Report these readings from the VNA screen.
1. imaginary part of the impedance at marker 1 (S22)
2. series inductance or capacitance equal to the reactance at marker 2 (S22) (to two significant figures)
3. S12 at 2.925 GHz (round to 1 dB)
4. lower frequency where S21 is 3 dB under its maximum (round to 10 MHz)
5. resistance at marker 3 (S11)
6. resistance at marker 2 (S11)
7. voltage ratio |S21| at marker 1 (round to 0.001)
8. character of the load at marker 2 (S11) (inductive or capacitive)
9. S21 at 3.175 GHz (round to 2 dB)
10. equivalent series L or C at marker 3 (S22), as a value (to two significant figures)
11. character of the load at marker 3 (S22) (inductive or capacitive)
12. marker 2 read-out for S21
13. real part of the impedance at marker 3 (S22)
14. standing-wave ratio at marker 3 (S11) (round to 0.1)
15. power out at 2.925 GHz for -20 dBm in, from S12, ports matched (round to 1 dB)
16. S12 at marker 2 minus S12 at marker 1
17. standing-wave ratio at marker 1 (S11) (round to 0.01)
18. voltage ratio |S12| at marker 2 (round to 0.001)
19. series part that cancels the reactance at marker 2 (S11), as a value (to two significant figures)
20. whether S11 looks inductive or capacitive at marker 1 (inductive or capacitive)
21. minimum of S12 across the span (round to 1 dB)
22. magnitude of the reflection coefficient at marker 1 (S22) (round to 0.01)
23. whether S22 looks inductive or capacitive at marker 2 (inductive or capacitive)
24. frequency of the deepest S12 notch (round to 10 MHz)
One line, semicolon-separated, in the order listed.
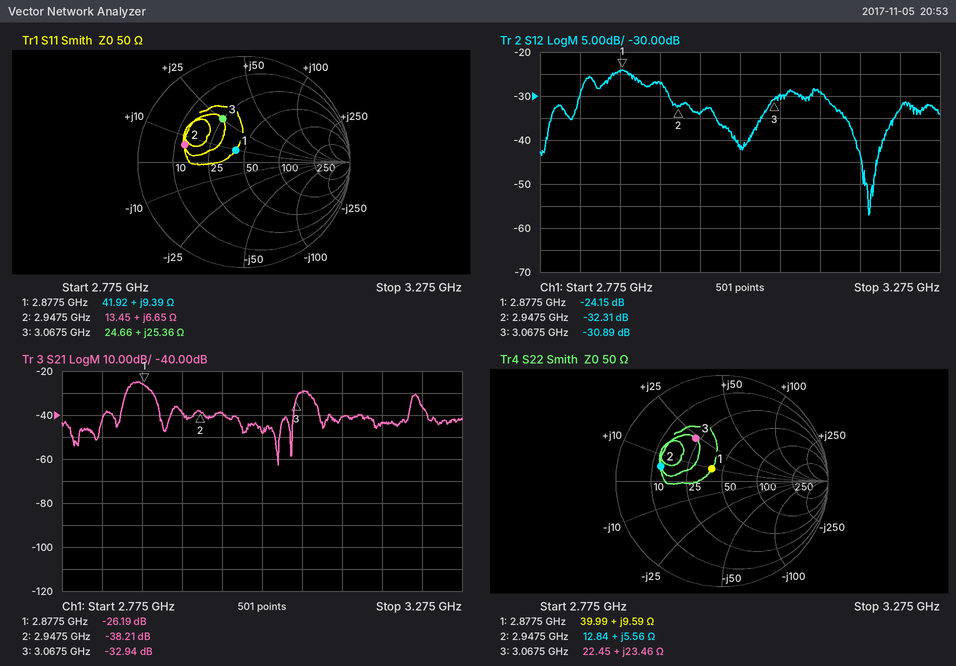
+9.59 Ω; 300 pH; -27 dB; 2.86 GHz; 24.66 Ω; 13.45 Ω; 0.049; inductive; -44 dB; 1.2 nH; inductive; -38.21 dB; 22.45 Ω; 2.7; -47 dBm; -8.16 dB; 1.31; 0.024; 8.1 pF; inductive; -57 dB; 0.15; inductive; 3.19 GHz
